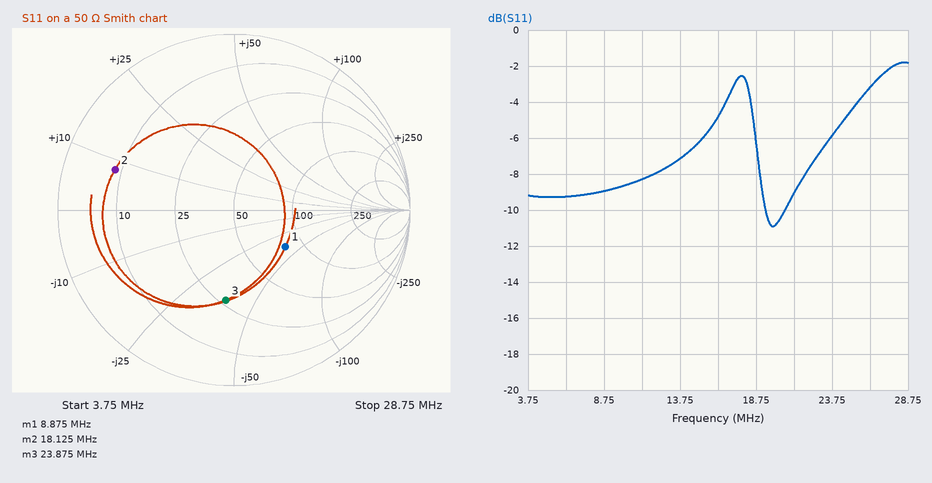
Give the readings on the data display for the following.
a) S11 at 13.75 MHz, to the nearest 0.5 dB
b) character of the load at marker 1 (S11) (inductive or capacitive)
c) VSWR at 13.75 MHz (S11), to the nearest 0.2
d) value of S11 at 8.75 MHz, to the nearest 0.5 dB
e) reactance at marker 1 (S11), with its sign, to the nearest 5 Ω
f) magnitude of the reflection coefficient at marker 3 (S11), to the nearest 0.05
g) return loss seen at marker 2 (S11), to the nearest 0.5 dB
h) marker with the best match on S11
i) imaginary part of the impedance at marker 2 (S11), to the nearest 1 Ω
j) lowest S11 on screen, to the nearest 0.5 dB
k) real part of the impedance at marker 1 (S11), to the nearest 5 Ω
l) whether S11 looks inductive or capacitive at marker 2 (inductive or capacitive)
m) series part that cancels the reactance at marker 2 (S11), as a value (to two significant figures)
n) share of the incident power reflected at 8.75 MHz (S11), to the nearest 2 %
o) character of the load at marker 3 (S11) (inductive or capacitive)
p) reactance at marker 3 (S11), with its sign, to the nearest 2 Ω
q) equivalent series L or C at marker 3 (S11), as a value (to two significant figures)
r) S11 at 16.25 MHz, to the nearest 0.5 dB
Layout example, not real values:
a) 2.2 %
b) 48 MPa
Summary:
a) -7.0 dB
b) capacitive
c) 2.6
d) -9.0 dB
e) -40 Ω
f) 0.50
g) 3.0 dB
h) marker 1
i) +8 Ω
j) -11.0 dB
k) 80 Ω
l) inductive
m) 1.1 nF
n) 12 %
o) capacitive
p) -38 Ω
q) 180 pF
r) -5.0 dB
